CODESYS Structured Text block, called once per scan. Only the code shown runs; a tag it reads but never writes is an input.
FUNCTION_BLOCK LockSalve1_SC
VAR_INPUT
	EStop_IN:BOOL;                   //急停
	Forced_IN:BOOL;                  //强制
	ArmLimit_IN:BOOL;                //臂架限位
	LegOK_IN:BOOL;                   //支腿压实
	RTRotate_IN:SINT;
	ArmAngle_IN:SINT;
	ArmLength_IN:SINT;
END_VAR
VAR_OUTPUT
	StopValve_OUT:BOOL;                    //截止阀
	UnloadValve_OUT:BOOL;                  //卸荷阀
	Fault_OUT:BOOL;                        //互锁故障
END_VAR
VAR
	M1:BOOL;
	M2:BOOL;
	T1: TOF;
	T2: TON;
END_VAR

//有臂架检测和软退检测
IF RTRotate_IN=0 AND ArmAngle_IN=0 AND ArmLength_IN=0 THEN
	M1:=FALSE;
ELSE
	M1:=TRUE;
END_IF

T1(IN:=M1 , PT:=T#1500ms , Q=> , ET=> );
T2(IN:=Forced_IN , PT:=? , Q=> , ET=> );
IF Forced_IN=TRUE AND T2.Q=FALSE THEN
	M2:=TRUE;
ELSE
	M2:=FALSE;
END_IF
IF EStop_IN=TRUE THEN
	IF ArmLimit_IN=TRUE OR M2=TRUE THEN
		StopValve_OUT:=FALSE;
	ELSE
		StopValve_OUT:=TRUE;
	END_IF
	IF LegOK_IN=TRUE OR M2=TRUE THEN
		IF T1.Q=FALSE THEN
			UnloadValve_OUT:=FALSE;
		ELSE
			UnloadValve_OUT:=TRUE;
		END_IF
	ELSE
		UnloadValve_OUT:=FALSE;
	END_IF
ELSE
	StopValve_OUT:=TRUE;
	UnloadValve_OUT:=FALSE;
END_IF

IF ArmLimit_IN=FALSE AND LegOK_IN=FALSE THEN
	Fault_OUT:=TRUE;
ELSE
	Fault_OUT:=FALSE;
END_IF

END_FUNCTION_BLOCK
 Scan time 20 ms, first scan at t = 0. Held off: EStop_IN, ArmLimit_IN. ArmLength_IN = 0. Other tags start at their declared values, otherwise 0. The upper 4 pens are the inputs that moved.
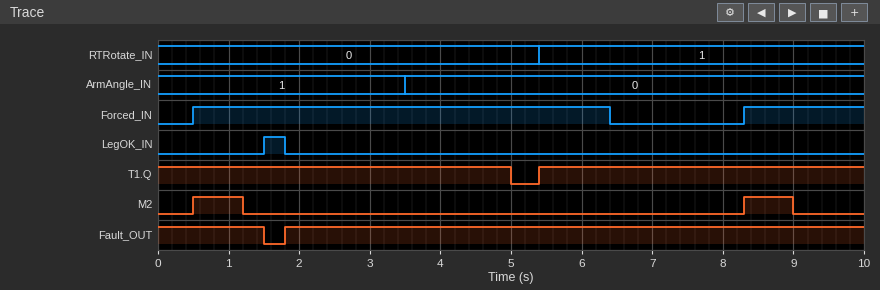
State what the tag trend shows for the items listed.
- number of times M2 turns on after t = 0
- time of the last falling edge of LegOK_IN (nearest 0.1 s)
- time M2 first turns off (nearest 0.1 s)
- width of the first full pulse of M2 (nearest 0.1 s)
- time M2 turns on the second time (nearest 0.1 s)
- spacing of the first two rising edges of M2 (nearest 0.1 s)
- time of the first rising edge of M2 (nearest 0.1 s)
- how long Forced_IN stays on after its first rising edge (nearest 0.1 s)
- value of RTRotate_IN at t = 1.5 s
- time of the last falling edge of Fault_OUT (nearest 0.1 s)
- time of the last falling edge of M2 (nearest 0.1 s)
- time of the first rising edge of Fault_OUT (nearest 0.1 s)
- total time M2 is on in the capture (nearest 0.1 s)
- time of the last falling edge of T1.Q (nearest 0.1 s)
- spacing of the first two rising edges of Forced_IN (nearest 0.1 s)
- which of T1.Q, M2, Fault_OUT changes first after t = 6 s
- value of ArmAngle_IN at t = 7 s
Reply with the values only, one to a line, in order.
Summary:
2
1.8 s
1.2 s
0.7 s
8.3 s
7.8 s
0.5 s
5.9 s
0
1.5 s
9.0 s
1.8 s
1.4 s
5.0 s
7.8 s
M2
0
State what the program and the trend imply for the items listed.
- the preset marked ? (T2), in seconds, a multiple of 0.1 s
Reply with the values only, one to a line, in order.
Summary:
0.7 s
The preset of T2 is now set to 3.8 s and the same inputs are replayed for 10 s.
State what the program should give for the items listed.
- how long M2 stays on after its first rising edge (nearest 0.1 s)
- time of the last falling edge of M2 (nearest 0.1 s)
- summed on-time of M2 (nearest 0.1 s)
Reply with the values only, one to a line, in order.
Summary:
3.8 s
4.3 s
5.5 s
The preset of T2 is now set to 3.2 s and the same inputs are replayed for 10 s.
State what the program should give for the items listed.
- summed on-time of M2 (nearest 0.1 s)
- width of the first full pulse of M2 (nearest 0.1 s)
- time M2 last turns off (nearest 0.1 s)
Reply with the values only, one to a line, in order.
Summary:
4.9 s
3.2 s
3.7 s
